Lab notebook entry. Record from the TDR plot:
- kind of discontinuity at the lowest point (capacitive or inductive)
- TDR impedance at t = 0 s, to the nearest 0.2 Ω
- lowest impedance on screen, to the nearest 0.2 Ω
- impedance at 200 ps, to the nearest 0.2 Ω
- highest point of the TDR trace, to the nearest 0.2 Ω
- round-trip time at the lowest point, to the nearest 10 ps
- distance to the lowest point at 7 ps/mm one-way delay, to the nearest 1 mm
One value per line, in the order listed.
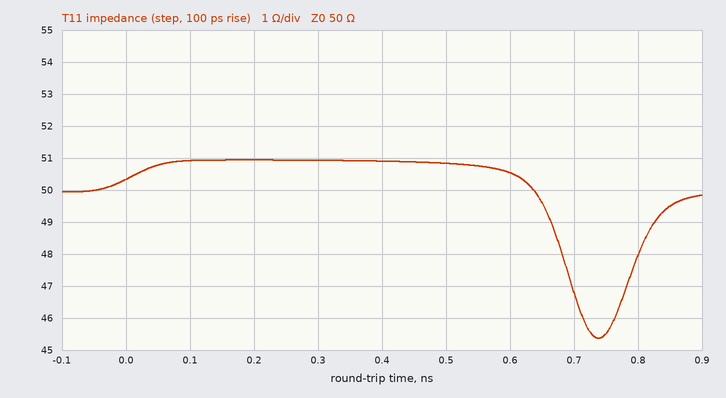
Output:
capacitive
50.4 Ω
45.4 Ω
51.0 Ω
51.0 Ω
740 ps
53 mm
